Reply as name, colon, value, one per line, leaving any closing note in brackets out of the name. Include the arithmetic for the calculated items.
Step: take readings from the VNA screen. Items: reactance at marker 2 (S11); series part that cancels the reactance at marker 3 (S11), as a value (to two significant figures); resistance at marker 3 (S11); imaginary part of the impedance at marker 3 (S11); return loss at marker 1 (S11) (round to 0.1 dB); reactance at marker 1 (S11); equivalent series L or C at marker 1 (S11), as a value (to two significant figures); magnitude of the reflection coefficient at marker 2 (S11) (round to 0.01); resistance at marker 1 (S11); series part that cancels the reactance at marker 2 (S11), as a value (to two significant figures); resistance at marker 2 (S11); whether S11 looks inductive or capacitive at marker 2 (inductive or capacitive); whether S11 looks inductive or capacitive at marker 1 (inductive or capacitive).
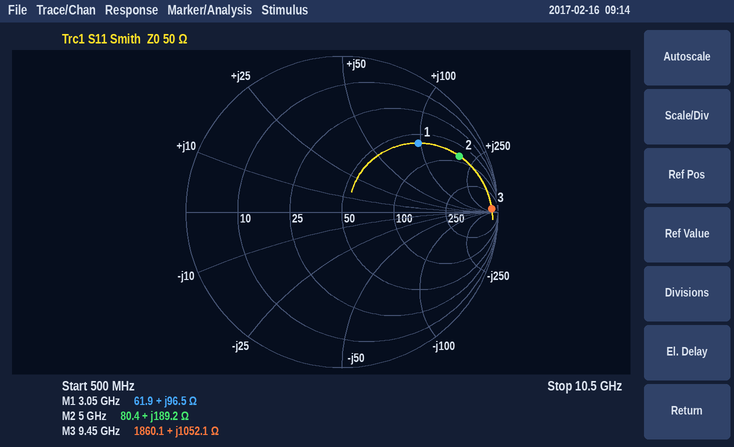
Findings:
reactance at marker 2: +189.2 Ω
series part that cancels the reactance at marker 3 (S11), as a value: C = 1/(2π × 9.45 GHz × 1052.1 Ω) ≈ 16 fF
resistance at marker 3: 1860.1 Ω
imaginary part of the impedance at marker 3: +1052.1 Ω
return loss at marker 1 (S11): 3.6 dB
reactance at marker 1: +96.5 Ω
equivalent series L or C at marker 1 (S11), as a value: L = 96.5 Ω/(2π × 3.05 GHz) ≈ 5.0 nH
magnitude of the reflection coefficient at marker 2 (S11): 0.83
resistance at marker 1: 61.9 Ω
series part that cancels the reactance at marker 2 (S11), as a value: C = 1/(2π × 5 GHz × 189.2 Ω) ≈ 168 fF, so 170 fF to two significant figures
resistance at marker 2: 80.4 Ω
whether S11 looks inductive or capacitive at marker 2: inductive
whether S11 looks inductive or capacitive at marker 1: inductive
